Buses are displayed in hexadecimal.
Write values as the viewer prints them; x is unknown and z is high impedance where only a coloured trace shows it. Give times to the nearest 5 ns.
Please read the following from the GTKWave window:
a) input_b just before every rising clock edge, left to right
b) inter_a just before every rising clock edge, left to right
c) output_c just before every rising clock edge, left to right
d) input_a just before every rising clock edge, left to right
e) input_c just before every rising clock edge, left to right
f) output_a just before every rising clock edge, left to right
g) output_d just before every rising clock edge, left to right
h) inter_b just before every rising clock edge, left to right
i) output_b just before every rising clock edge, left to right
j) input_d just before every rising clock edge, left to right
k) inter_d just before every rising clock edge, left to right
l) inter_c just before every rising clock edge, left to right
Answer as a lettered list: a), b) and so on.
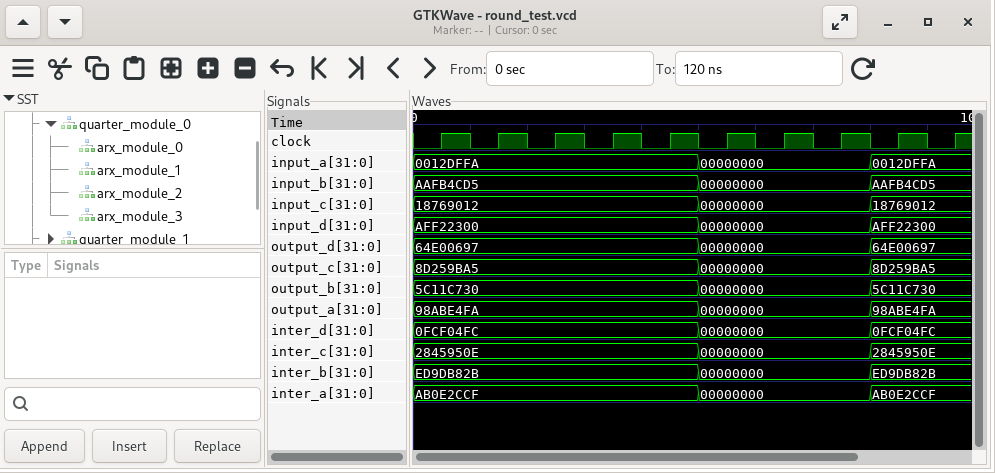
a) AAFB4CD5, AAFB4CD5, AAFB4CD5, AAFB4CD5, AAFB4CD5, 00000000, 00000000, 00000000, AAFB4CD5, AAFB4CD5
b) AB0E2CCF, AB0E2CCF, AB0E2CCF, AB0E2CCF, AB0E2CCF, 00000000, 00000000, 00000000, AB0E2CCF, AB0E2CCF
c) 8D259BA5, 8D259BA5, 8D259BA5, 8D259BA5, 8D259BA5, 00000000, 00000000, 00000000, 8D259BA5, 8D259BA5
d) 0012DFFA, 0012DFFA, 0012DFFA, 0012DFFA, 0012DFFA, 00000000, 00000000, 00000000, 0012DFFA, 0012DFFA
e) 18769012, 18769012, 18769012, 18769012, 18769012, 00000000, 00000000, 00000000, 18769012, 18769012
f) 98ABE4FA, 98ABE4FA, 98ABE4FA, 98ABE4FA, 98ABE4FA, 00000000, 00000000, 00000000, 98ABE4FA, 98ABE4FA
g) 64E00697, 64E00697, 64E00697, 64E00697, 64E00697, 00000000, 00000000, 00000000, 64E00697, 64E00697
h) ED9DB82B, ED9DB82B, ED9DB82B, ED9DB82B, ED9DB82B, 00000000, 00000000, 00000000, ED9DB82B, ED9DB82B
i) 5C11C730, 5C11C730, 5C11C730, 5C11C730, 5C11C730, 00000000, 00000000, 00000000, 5C11C730, 5C11C730
j) AFF22300, AFF22300, AFF22300, AFF22300, AFF22300, 00000000, 00000000, 00000000, AFF22300, AFF22300
k) 0FCF04FC, 0FCF04FC, 0FCF04FC, 0FCF04FC, 0FCF04FC, 00000000, 00000000, 00000000, 0FCF04FC, 0FCF04FC
l) 2845950E, 2845950E, 2845950E, 2845950E, 2845950E, 00000000, 00000000, 00000000, 2845950E, 2845950E
